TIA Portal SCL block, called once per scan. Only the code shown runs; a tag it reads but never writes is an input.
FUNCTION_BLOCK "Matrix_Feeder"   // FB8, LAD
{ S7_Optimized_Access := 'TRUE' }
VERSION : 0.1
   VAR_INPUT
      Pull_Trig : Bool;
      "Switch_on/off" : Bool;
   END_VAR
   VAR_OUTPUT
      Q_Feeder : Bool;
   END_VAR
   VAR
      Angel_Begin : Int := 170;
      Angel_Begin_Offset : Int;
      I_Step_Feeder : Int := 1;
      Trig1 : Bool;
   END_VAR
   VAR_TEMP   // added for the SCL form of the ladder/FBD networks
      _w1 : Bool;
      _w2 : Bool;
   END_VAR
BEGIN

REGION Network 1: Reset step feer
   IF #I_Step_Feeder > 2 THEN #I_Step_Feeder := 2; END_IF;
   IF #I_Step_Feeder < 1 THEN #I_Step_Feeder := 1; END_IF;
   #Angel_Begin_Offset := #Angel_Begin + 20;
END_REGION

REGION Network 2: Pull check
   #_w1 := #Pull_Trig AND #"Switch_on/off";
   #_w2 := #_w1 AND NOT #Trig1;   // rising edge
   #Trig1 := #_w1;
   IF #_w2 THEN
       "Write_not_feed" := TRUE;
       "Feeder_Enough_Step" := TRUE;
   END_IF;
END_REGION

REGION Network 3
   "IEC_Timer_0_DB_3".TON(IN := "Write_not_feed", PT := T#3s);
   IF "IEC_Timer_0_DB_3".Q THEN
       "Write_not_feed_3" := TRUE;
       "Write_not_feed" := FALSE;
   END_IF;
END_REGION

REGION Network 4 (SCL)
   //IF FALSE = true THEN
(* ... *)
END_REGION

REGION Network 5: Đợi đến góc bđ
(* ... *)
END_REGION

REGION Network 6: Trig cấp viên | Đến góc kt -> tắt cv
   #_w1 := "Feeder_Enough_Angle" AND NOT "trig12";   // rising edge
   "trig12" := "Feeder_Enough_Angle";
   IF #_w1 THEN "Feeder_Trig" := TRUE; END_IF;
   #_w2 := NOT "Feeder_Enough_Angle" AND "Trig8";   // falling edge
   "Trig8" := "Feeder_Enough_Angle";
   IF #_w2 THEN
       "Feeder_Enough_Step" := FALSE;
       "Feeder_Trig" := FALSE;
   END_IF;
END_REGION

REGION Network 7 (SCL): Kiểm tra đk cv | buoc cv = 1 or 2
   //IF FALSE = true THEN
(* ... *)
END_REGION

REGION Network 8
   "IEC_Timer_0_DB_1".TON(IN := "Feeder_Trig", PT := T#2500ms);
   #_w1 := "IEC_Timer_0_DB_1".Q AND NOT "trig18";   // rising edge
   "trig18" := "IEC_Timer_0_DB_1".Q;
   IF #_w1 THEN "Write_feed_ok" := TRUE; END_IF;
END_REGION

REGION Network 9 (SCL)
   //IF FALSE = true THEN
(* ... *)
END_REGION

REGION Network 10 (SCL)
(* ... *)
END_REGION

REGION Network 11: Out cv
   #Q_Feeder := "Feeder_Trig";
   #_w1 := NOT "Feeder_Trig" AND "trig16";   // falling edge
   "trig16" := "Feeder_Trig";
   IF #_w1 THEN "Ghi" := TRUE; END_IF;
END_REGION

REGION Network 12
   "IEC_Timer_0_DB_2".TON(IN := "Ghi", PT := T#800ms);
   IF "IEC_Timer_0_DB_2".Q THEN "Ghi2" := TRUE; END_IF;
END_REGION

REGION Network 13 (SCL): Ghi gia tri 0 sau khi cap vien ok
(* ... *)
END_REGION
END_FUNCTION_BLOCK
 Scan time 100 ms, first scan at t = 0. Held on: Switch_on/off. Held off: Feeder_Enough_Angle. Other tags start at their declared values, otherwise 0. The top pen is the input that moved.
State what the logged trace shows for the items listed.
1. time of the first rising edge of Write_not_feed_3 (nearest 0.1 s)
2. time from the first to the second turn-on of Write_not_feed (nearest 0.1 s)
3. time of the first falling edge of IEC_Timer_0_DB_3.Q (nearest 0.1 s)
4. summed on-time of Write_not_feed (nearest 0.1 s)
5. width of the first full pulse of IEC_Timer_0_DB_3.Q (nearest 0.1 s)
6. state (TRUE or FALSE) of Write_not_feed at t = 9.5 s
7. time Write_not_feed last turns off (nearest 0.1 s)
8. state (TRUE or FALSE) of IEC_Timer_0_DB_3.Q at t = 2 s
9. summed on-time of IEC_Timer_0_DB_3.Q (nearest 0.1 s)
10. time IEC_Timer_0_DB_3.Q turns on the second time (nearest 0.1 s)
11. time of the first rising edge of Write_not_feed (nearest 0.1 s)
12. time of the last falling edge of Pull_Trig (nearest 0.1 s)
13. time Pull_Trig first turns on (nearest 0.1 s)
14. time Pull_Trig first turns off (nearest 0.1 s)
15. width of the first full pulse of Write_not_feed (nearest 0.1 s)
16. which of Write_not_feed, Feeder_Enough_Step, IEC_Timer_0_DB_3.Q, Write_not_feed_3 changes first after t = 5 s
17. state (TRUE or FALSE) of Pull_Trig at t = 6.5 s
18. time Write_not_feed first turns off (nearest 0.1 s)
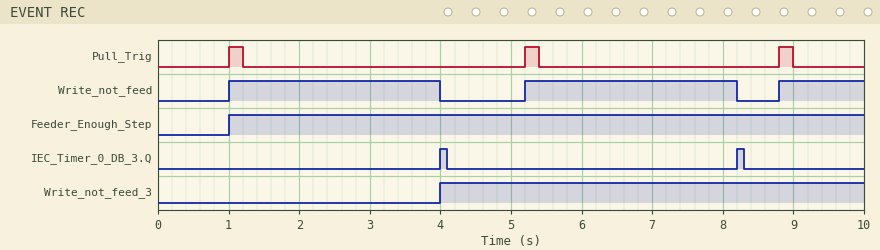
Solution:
4.0 s
4.2 s
4.1 s
7.2 s
0.1 s
TRUE
8.2 s
FALSE
0.2 s
8.2 s
1.0 s
9.0 s
1.0 s
1.2 s
3.0 s
Write_not_feed
FALSE
4.0 s
